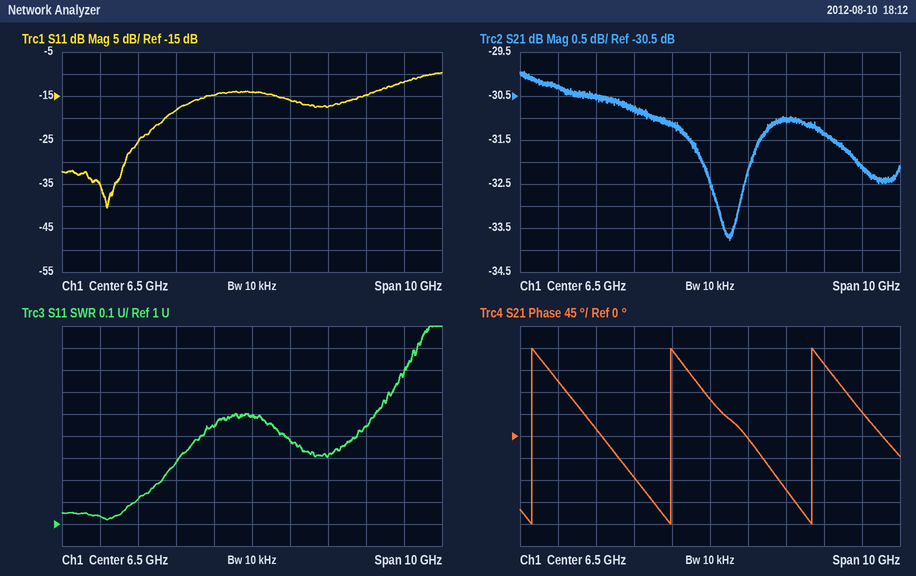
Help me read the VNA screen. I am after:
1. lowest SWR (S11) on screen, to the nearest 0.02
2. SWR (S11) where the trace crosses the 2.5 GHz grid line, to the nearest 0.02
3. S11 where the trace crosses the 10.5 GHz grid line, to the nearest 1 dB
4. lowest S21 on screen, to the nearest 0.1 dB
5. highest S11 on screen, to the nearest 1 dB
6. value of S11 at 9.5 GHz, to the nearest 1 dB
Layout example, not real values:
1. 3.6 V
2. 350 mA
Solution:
1. 1.02
2. 1.04
3. -12 dB
4. -33.8 dB
5. -10 dB
6. -15 dB
